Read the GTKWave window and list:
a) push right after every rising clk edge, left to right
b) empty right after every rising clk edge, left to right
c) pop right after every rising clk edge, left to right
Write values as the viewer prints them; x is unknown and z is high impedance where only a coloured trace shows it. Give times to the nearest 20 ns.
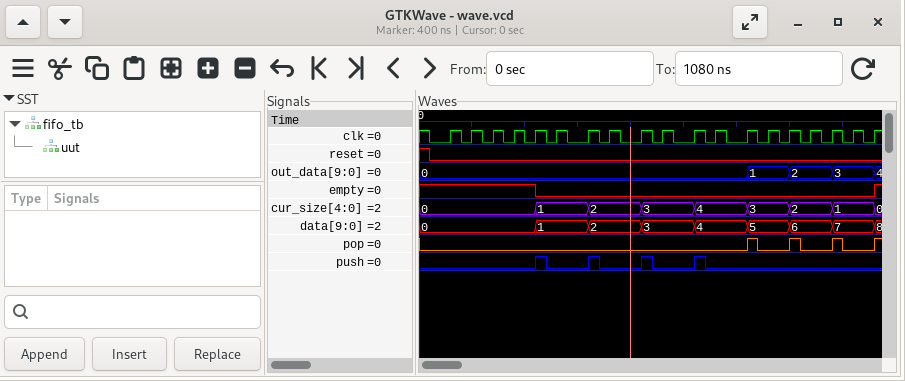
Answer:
0 0 0 0 1 0 1 0 1 0 1 0 0 0 0 0 0 0 0
1 1 1 1 0 0 0 0 0 0 0 0 0 0 0 0 0 0 1
0 0 0 0 0 0 0 0 0 0 0 0 1 0 1 0 1 0 1
